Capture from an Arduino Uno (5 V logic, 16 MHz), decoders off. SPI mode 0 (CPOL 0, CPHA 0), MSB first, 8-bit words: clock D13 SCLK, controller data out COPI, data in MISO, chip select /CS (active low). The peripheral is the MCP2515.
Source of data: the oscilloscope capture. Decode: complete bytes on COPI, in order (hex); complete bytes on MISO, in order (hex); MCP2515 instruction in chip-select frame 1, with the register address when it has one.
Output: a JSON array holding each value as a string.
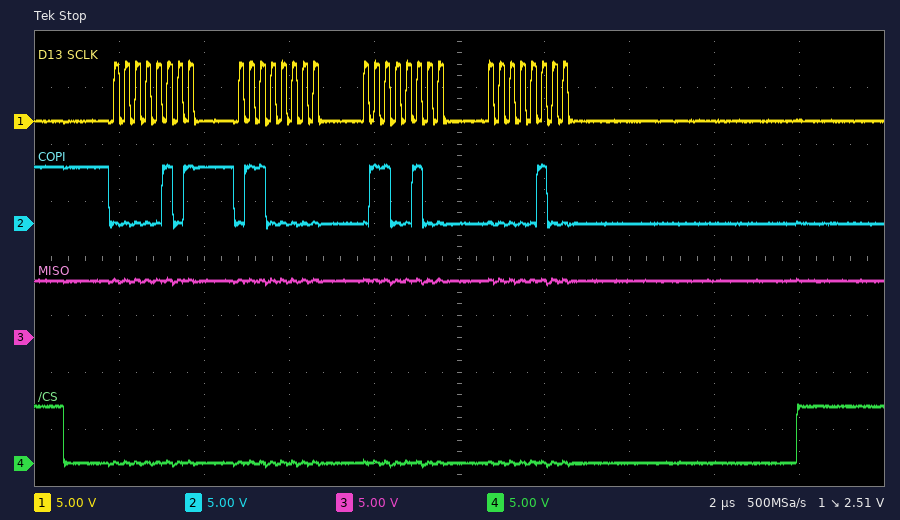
["05 60 64 04", "FF FF FF FF", "BIT MODIFY 0x60"]
